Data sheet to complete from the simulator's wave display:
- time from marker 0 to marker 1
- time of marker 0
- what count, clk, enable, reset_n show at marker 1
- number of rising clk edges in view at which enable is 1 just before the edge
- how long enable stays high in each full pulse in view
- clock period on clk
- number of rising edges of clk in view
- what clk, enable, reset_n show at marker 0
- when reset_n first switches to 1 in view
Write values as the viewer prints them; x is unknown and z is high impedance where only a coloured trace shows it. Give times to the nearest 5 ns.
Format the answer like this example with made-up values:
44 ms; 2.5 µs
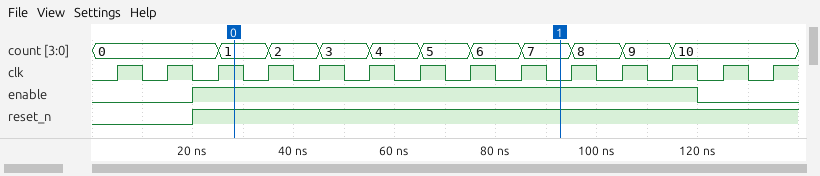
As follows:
65 ns; 30 ns; count=7, clk=0, enable=1, reset_n=1; 10; 100 ns; 10 ns; 14; clk=1, enable=1, reset_n=1; 20 ns
